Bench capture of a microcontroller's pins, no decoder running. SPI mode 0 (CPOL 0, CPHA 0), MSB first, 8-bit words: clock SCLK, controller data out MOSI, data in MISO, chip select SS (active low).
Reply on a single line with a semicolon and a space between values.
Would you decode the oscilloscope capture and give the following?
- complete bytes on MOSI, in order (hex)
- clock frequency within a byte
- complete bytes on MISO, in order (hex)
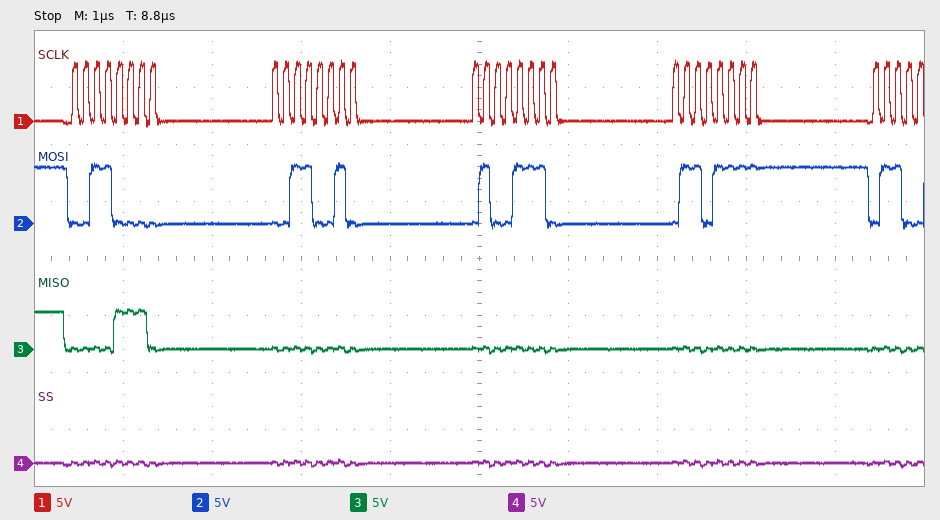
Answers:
30 32 4E 6F; 8 MHz; 0E 00 00 00
